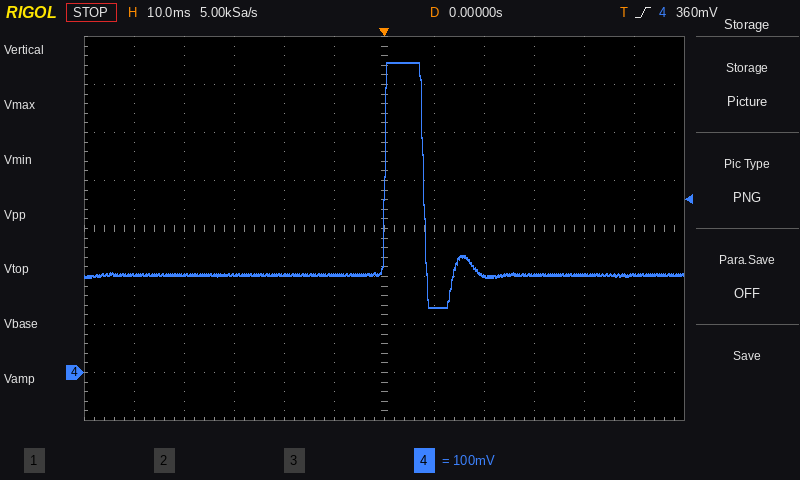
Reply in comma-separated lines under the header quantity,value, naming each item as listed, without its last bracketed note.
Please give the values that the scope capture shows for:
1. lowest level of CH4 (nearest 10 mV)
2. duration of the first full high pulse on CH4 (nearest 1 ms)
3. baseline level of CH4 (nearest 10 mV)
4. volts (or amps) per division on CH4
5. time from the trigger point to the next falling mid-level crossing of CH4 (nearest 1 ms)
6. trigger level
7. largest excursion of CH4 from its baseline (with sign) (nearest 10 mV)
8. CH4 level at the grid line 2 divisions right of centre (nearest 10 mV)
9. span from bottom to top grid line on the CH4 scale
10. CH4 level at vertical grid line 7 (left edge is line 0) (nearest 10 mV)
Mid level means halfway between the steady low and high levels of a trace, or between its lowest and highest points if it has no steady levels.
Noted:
quantity,value
lowest level of CH4,140 mV
duration of the first full high pulse on CH4,8 ms
baseline level of CH4,200 mV
volts (or amps) per division on CH4,100 mV
time from the trigger point to the next falling mid-level crossing of CH4,8 ms
trigger level,360 mV
largest excursion of CH4 from its baseline (with sign),+440 mV
CH4 level at the grid line 2 divisions right of centre,200 mV
span from bottom to top grid line on the CH4 scale,800 mV
CH4 level at vertical grid line 7 (left edge is line 0),140 mV
